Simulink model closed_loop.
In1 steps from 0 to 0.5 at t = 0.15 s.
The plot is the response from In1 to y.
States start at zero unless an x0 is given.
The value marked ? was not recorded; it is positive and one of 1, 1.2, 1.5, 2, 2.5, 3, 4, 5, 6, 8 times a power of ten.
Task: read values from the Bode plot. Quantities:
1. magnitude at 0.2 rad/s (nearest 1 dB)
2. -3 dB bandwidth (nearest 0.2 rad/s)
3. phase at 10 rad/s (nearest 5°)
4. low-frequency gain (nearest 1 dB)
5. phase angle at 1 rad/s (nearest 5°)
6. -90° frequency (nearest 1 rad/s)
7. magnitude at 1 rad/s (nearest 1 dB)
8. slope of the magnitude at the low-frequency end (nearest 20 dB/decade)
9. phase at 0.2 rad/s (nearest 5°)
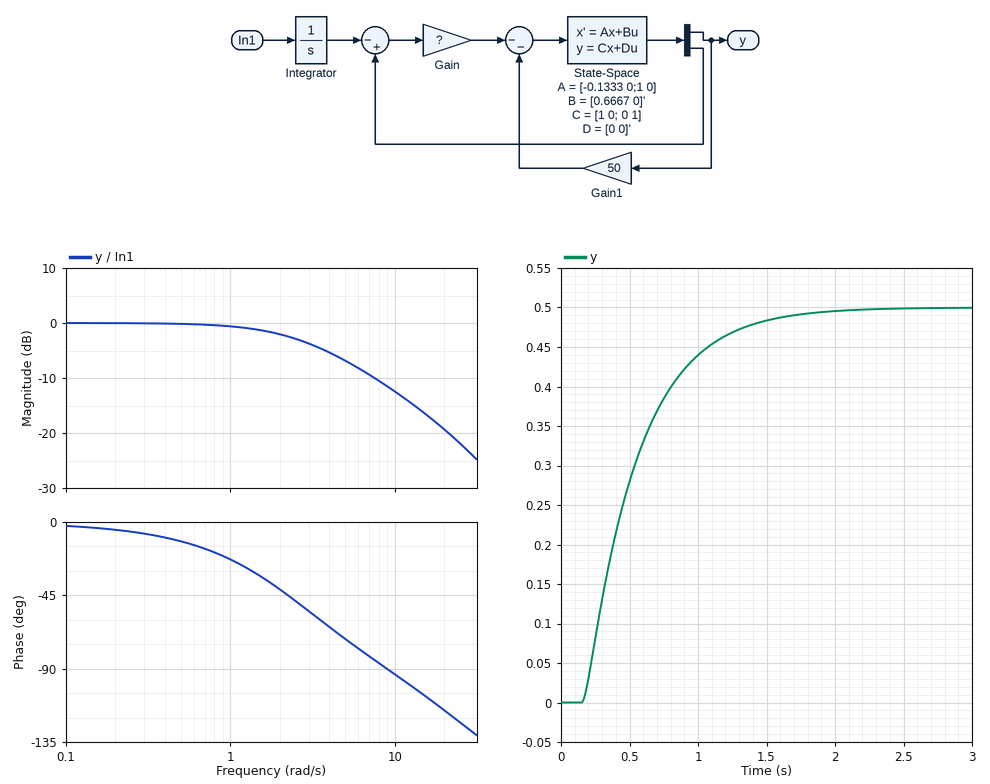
0 dB
2.6 rad/s
-95°
0 dB
-25°
9 rad/s
-1 dB
0 dB/decade
-5°
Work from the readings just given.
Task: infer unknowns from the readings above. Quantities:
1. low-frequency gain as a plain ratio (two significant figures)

1.0
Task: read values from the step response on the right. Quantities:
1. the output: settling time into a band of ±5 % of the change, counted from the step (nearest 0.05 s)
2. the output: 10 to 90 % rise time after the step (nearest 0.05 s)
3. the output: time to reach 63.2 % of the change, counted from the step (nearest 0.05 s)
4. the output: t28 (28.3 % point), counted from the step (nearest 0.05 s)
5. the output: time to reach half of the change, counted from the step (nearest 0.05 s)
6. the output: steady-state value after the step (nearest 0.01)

1.20 s
0.85 s
0.40 s
0.15 s
0.30 s
0.50
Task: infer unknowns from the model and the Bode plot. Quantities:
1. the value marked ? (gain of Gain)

120
